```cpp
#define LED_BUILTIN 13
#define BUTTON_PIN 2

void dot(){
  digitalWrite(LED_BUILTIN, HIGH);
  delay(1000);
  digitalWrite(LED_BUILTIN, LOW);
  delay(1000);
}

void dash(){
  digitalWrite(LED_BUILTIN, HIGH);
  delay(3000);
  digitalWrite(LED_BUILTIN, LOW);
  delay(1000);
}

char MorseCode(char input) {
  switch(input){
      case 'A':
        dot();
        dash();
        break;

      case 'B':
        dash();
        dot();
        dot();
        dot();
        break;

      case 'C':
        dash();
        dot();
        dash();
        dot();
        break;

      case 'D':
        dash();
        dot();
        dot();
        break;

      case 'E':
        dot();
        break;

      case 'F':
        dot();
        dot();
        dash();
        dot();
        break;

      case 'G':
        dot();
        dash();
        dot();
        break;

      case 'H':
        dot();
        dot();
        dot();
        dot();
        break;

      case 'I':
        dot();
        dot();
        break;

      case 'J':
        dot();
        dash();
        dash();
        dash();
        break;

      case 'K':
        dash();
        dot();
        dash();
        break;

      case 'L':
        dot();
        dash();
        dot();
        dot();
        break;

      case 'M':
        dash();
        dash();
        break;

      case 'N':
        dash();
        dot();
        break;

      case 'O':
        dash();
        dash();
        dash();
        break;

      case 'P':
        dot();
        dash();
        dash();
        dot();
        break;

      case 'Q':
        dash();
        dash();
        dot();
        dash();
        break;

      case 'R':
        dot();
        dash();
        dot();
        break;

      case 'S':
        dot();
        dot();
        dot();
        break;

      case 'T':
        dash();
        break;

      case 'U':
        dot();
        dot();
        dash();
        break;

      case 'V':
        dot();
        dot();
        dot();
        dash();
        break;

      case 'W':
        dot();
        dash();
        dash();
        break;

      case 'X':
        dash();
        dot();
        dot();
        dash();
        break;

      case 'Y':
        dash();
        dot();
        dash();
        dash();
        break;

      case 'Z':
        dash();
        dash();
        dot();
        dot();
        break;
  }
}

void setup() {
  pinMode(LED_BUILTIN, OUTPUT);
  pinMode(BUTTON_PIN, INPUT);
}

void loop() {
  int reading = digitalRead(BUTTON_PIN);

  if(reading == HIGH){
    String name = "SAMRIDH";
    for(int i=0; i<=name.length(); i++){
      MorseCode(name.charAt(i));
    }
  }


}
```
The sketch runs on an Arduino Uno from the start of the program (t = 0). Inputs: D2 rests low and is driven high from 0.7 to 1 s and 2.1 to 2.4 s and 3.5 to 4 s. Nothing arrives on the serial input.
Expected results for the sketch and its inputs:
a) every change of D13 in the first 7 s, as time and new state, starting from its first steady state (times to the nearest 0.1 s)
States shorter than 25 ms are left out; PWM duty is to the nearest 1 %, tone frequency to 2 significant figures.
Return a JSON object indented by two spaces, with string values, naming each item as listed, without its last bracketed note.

{
  "every change of D13 in the first 7 s, as time and new state, starting from its first steady state": "0 s low; 0.7 s high; 1.7 s low; 2.7 s high; 3.7 s low; 4.7 s high; 5.7 s low; 6.7 s high"
}
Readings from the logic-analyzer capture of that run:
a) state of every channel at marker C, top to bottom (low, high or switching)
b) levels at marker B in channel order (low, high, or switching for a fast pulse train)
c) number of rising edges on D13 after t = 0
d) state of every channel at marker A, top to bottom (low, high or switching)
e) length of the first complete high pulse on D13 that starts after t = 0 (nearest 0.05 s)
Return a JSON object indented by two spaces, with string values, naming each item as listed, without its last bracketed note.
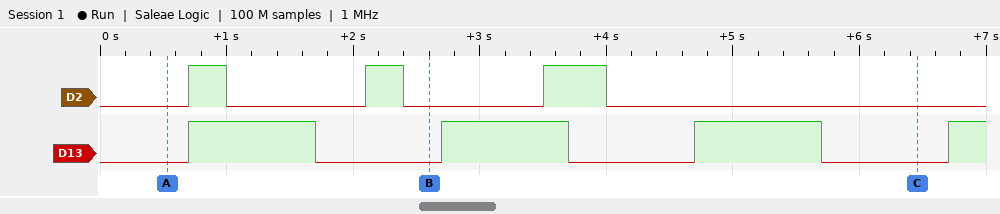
{
  "state of every channel at marker C, top to bottom": "D2 low, D13 low",
  "levels at marker B in channel order": "D2 low, D13 low",
  "number of rising edges on D13 after t = 0": "4",
  "state of every channel at marker A, top to bottom": "D2 low, D13 low",
  "length of the first complete high pulse on D13 that starts after t = 0": "1.00 s"
}
